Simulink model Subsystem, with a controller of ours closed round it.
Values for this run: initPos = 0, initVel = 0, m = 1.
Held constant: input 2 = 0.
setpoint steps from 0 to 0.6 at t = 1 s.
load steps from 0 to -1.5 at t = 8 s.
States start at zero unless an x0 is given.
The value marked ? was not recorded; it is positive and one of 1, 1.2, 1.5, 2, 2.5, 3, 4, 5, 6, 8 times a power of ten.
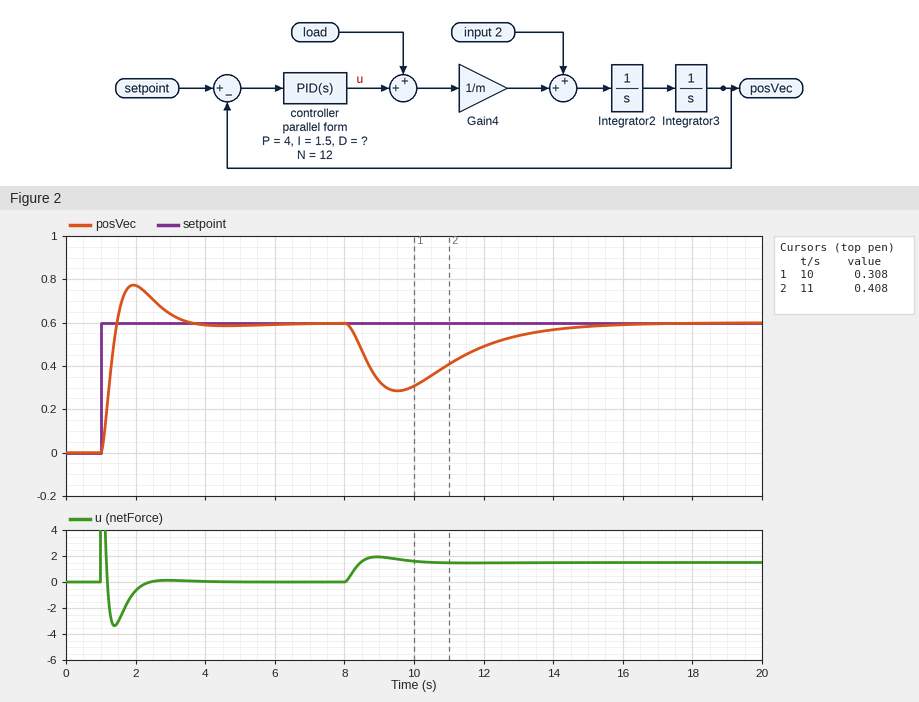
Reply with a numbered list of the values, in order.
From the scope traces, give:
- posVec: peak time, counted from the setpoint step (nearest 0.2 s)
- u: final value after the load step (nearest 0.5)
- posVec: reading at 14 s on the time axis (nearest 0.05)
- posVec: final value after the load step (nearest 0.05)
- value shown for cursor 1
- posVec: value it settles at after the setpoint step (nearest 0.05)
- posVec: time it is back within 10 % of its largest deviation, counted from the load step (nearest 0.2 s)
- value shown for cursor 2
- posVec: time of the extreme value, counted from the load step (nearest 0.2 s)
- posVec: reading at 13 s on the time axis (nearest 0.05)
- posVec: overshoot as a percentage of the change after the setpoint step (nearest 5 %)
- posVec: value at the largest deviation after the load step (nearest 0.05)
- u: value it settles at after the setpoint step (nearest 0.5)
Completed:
1. 1.0 s
2. 1.5
3. 0.55
4. 0.60
5. 0.308
6. 0.60
7. 6.0 s
8. 0.408
9. 1.6 s
10. 0.55
11. 30 %
12. 0.30
13. 0.0
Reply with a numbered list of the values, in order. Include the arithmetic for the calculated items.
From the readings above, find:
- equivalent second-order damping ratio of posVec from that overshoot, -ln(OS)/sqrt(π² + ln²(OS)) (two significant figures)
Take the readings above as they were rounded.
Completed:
1. ln(0.3) = -1.204; 1.204 / sqrt(9.870 + 1.450) = 0.36
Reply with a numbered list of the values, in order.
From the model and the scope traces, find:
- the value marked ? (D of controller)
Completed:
1. 3
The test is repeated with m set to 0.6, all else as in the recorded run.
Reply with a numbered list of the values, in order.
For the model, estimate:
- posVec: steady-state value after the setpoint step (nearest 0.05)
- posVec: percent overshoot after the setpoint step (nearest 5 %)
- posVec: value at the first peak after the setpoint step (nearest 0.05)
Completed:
1. 0.60
2. 25 %
3. 0.75
